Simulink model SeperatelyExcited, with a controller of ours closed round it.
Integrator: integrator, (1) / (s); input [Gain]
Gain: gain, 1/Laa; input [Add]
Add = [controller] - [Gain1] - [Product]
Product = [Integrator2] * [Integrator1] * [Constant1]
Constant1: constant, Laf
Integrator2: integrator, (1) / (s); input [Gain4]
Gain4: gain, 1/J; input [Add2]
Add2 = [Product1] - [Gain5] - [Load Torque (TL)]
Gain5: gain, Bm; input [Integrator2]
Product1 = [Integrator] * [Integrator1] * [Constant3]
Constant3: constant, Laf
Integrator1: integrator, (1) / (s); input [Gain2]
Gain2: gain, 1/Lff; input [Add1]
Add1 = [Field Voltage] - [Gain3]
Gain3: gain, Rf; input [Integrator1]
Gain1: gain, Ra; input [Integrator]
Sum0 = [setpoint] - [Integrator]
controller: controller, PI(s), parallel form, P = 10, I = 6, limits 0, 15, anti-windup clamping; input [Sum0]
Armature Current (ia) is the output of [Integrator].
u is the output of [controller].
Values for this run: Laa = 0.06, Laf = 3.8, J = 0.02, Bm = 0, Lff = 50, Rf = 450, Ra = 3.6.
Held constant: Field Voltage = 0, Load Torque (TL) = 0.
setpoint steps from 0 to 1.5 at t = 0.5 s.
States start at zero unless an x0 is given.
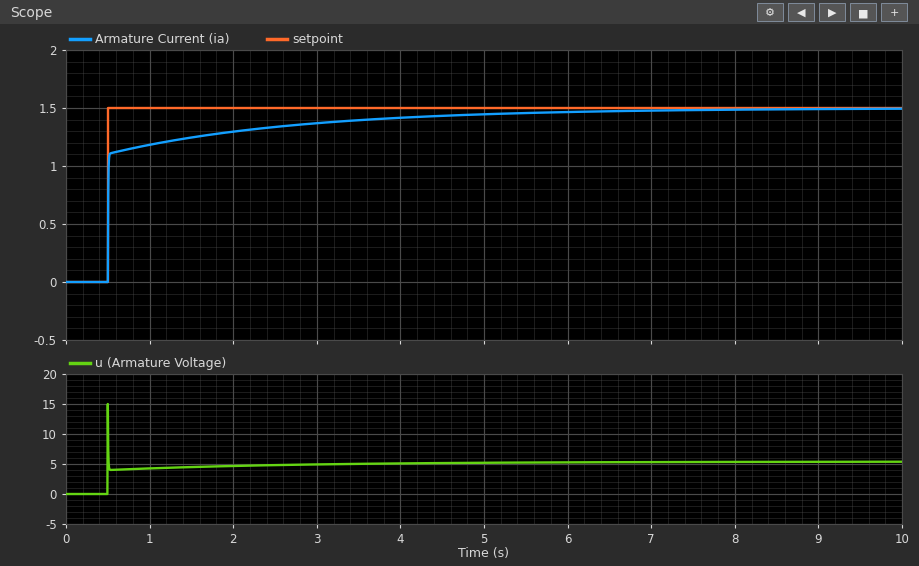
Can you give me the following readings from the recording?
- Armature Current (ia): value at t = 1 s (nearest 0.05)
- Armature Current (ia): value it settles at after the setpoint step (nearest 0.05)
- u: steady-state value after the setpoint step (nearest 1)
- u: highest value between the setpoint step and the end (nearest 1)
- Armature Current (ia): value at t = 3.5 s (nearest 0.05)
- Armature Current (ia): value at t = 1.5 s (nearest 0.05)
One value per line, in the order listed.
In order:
1.20
1.50
5
15
1.40
1.25
